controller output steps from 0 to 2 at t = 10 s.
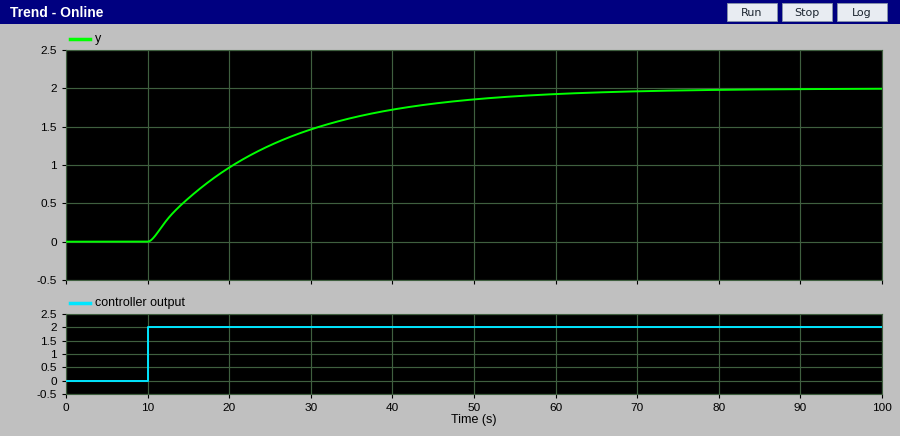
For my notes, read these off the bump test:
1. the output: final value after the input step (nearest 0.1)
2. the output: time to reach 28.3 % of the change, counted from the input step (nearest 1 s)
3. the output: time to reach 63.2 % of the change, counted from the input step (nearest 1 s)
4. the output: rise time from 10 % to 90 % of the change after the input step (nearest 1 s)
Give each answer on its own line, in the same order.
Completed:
2.0
5 s
15 s
33 s
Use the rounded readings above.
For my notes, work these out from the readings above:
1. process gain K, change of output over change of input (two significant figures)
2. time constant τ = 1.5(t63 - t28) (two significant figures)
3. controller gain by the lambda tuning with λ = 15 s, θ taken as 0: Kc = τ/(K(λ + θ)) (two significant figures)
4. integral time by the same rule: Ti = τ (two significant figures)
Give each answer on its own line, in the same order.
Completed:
1.0
15 s
1.0
15 s
